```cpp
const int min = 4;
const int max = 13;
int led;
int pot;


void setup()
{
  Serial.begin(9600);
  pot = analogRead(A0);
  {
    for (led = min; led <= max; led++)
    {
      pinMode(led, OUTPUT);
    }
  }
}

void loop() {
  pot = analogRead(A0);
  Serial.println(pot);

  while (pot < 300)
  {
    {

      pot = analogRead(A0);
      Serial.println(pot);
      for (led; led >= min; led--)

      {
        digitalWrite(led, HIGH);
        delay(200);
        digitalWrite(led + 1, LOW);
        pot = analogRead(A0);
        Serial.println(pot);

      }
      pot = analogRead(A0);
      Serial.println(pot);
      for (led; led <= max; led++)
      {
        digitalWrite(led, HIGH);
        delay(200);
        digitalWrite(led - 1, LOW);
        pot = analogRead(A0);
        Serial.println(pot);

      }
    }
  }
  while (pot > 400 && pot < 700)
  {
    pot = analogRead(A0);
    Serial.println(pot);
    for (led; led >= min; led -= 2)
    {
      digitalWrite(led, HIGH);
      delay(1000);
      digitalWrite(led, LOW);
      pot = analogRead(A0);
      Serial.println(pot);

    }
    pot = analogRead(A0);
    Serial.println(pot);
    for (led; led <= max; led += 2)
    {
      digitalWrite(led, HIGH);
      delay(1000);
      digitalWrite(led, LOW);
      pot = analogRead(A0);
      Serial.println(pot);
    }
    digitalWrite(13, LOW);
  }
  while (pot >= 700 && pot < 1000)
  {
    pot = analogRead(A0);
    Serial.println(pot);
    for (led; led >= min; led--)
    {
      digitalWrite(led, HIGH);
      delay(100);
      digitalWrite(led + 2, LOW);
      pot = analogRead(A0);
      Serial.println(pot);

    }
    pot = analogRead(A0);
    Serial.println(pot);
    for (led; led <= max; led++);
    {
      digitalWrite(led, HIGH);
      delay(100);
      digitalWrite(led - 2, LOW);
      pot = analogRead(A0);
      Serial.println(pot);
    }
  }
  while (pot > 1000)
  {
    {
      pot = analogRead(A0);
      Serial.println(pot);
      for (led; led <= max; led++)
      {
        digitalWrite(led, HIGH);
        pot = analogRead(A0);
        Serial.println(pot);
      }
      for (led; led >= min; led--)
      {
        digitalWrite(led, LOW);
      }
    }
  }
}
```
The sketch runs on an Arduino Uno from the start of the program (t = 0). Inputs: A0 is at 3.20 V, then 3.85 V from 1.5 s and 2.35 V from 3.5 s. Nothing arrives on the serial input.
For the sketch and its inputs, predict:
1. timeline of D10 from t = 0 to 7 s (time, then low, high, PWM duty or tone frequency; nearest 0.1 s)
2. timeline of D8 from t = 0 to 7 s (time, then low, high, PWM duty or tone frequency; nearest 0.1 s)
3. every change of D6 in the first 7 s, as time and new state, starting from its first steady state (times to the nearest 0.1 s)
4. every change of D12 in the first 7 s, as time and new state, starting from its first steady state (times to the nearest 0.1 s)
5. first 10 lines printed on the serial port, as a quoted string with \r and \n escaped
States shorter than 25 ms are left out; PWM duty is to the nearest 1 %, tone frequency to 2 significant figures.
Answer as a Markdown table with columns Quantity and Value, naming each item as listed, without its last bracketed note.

| Quantity | Value |
|---|---|
| timeline of D10 from t = 0 to 7 s | 0 s low; 2 s high; 3 s low |
| timeline of D8 from t = 0 to 7 s | 0 s low; 3 s high; 4 s low |
| every change of D6 in the first 7 s, as time and new state, starting from its first steady state | 0 s low; 4 s high; 5 s low |
| every change of D12 in the first 7 s, as time and new state, starting from its first steady state | 0 s low; 1 s high; 2 s low |
| first 10 lines printed on the serial port, as a quoted string with \r and \n escaped | "655\r\n655\r\n655\r\n788\r\n788\r\n481\r\n481\r\n481\r\n481\r\n481\r\n" |
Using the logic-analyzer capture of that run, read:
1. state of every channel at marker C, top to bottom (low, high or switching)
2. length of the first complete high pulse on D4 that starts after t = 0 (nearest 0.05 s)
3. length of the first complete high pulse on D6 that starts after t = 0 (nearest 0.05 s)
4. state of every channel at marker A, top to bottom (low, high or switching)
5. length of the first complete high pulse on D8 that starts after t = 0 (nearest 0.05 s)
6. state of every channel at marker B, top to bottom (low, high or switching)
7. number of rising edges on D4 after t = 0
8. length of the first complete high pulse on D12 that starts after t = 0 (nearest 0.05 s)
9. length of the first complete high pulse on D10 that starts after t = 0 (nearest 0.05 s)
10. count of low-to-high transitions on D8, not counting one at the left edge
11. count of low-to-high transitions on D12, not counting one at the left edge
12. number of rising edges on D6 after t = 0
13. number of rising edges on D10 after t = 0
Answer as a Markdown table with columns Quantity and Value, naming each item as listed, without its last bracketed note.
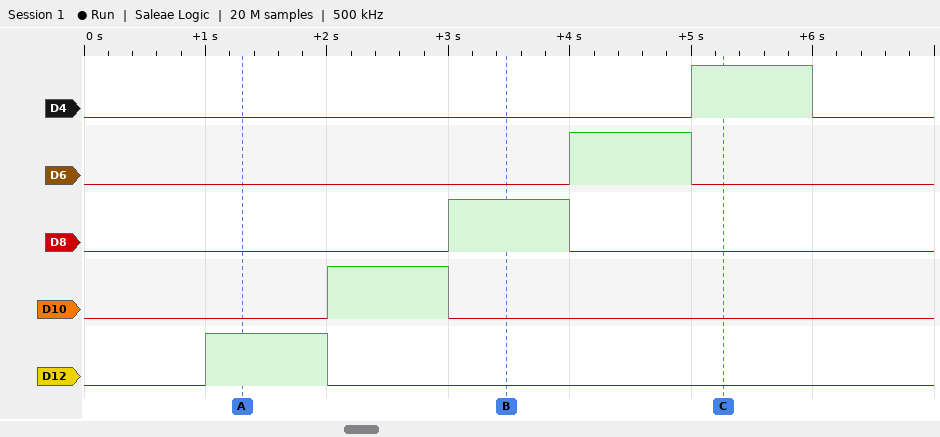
| Quantity | Value |
|---|---|
| state of every channel at marker C, top to bottom | D4 high, D6 low, D8 low, D10 low, D12 low |
| length of the first complete high pulse on D4 that starts after t = 0 | 1.00 s |
| length of the first complete high pulse on D6 that starts after t = 0 | 1.00 s |
| state of every channel at marker A, top to bottom | D4 low, D6 low, D8 low, D10 low, D12 high |
| length of the first complete high pulse on D8 that starts after t = 0 | 1.00 s |
| state of every channel at marker B, top to bottom | D4 low, D6 low, D8 high, D10 low, D12 low |
| number of rising edges on D4 after t = 0 | 1 |
| length of the first complete high pulse on D12 that starts after t = 0 | 1.00 s |
| length of the first complete high pulse on D10 that starts after t = 0 | 1.00 s |
| count of low-to-high transitions on D8, not counting one at the left edge | 1 |
| count of low-to-high transitions on D12, not counting one at the left edge | 1 |
| number of rising edges on D6 after t = 0 | 1 |
| number of rising edges on D10 after t = 0 | 1 |
